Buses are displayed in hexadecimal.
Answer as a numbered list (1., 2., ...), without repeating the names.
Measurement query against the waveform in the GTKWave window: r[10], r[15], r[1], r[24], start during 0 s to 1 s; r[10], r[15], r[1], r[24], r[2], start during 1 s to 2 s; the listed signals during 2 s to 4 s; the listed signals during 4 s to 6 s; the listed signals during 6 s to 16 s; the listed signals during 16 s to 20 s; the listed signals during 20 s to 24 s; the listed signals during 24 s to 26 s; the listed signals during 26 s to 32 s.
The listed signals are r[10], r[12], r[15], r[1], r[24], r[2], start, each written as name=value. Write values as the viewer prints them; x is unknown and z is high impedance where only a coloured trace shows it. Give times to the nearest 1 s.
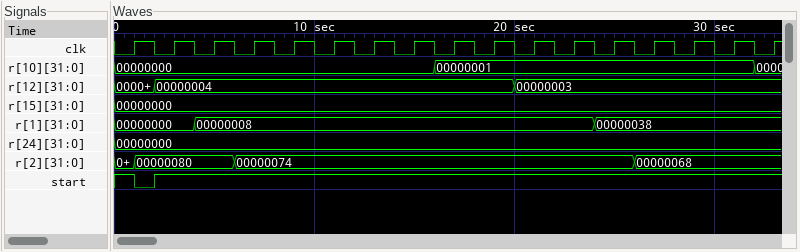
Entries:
1. r[10]=00000000, r[15]=00000000, r[1]=00000000, r[24]=00000000, start=1
2. r[10]=00000000, r[15]=00000000, r[1]=00000000, r[24]=00000000, r[2]=00000080, start=0
3. r[10]=00000000, r[12]=00000004, r[15]=00000000, r[1]=00000000, r[24]=00000000, r[2]=00000080, start=1
4. r[10]=00000000, r[12]=00000004, r[15]=00000000, r[1]=00000008, r[24]=00000000, r[2]=00000080, start=1
5. r[10]=00000000, r[12]=00000004, r[15]=00000000, r[1]=00000008, r[24]=00000000, r[2]=00000074, start=1
6. r[10]=00000001, r[12]=00000004, r[15]=00000000, r[1]=00000008, r[24]=00000000, r[2]=00000074, start=1
7. r[10]=00000001, r[12]=00000003, r[15]=00000000, r[1]=00000008, r[24]=00000000, r[2]=00000074, start=1
8. r[10]=00000001, r[12]=00000003, r[15]=00000000, r[1]=00000038, r[24]=00000000, r[2]=00000074, start=1
9. r[10]=00000001, r[12]=00000003, r[15]=00000000, r[1]=00000038, r[24]=00000000, r[2]=00000068, start=1
